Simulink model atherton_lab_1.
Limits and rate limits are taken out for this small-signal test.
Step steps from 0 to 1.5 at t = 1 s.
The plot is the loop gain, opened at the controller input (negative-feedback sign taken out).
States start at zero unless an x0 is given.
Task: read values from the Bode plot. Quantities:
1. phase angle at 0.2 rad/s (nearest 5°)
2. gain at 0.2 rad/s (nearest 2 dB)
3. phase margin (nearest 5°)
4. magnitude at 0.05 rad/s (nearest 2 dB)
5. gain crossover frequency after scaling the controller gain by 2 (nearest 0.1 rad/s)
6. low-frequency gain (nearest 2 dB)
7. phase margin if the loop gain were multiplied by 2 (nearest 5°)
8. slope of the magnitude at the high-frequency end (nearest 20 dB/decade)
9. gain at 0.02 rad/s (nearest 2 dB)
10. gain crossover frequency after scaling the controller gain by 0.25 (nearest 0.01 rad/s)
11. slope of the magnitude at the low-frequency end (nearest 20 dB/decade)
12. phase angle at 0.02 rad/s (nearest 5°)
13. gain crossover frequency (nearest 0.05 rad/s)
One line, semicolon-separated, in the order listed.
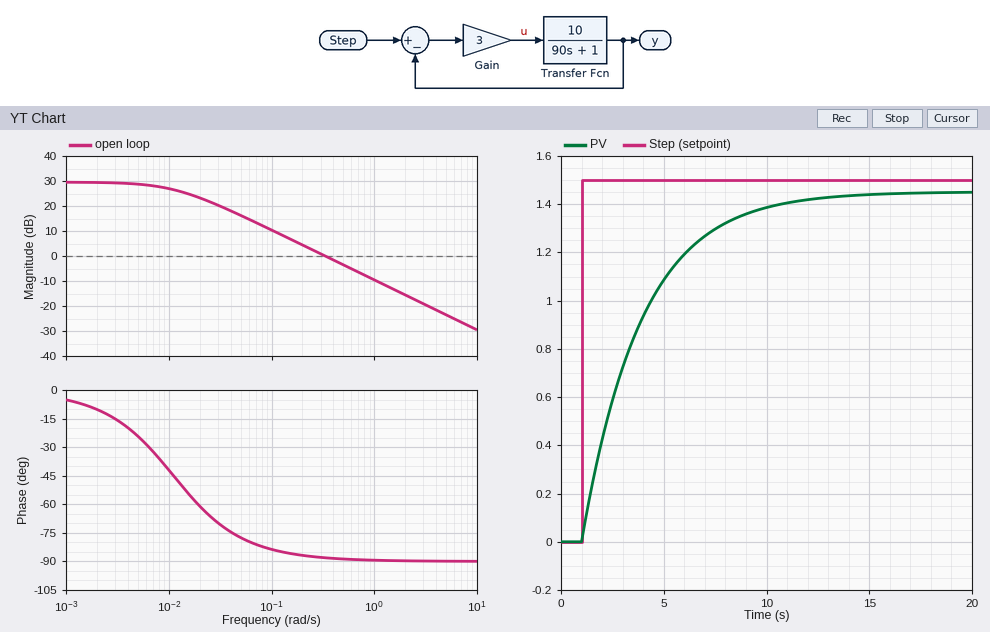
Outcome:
-85°; 4 dB; 90°; 16 dB; 0.7 rad/s; 30 dB; 90°; -20 dB/decade; 24 dB; 0.08 rad/s; 0 dB/decade; -60°; 0.35 rad/s
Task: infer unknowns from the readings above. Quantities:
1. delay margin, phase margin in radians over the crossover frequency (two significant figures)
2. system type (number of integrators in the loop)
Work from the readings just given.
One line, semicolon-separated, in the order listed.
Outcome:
4.5 s; 0
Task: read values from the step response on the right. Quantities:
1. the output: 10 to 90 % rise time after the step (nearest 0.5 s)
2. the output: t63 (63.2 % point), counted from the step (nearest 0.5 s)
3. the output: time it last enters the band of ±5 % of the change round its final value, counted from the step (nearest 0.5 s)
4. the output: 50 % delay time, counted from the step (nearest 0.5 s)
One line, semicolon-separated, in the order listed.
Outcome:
6.5 s; 3.0 s; 8.5 s; 2.0 s
